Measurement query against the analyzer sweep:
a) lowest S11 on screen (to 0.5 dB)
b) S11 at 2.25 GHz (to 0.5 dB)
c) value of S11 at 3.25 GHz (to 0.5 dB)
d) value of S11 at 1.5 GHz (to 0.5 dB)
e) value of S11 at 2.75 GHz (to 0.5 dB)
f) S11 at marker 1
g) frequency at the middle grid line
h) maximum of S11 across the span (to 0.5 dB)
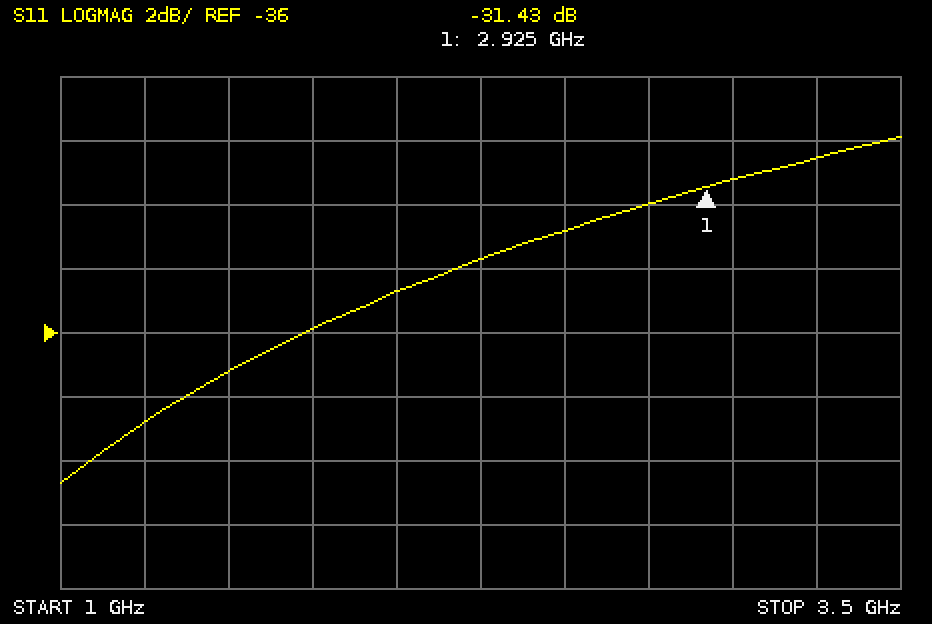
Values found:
-40.5 dB
-33.5 dB
-30.5 dB
-37.0 dB
-32.0 dB
-31.43 dB
2.25 GHz
-30.0 dB
